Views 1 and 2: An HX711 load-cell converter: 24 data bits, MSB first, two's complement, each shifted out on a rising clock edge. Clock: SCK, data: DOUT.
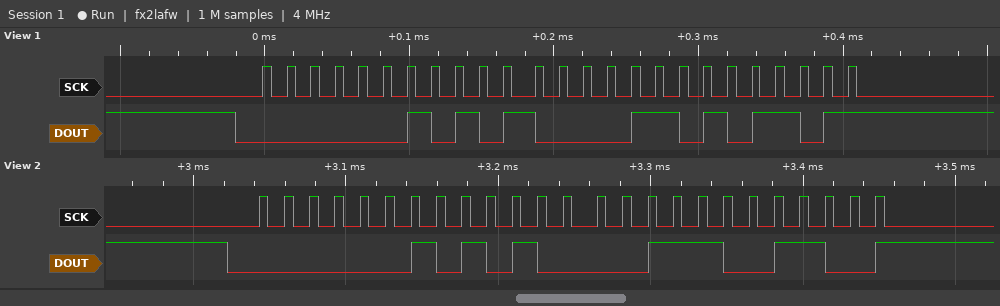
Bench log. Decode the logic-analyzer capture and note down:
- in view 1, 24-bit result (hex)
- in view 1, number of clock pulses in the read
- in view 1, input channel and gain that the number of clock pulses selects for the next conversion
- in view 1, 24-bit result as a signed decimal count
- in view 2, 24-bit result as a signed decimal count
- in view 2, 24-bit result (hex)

0x02A1AD
25
channel A, gain 128
172461
172492
0x02A1CC
